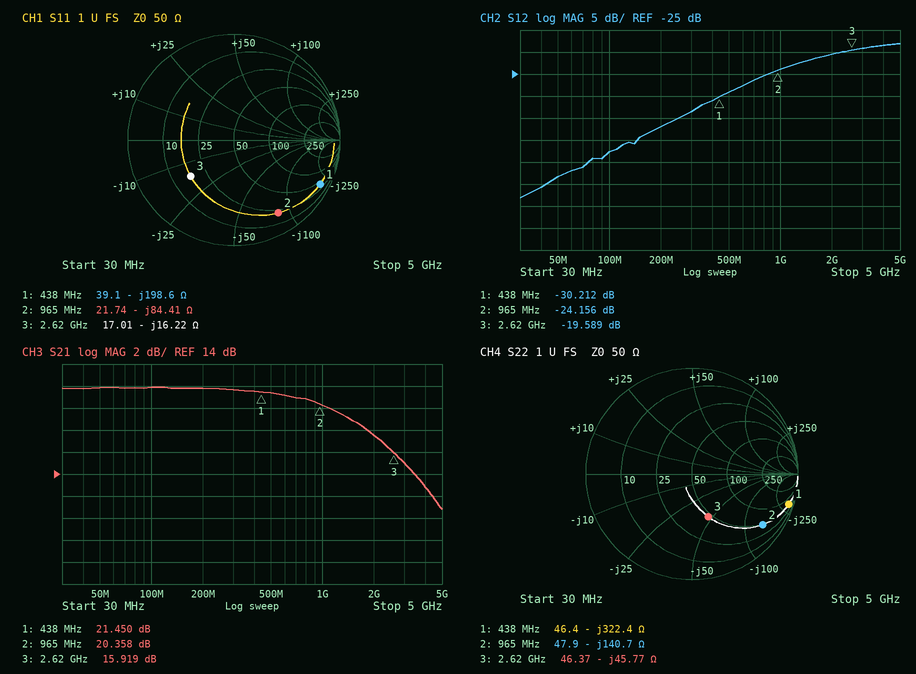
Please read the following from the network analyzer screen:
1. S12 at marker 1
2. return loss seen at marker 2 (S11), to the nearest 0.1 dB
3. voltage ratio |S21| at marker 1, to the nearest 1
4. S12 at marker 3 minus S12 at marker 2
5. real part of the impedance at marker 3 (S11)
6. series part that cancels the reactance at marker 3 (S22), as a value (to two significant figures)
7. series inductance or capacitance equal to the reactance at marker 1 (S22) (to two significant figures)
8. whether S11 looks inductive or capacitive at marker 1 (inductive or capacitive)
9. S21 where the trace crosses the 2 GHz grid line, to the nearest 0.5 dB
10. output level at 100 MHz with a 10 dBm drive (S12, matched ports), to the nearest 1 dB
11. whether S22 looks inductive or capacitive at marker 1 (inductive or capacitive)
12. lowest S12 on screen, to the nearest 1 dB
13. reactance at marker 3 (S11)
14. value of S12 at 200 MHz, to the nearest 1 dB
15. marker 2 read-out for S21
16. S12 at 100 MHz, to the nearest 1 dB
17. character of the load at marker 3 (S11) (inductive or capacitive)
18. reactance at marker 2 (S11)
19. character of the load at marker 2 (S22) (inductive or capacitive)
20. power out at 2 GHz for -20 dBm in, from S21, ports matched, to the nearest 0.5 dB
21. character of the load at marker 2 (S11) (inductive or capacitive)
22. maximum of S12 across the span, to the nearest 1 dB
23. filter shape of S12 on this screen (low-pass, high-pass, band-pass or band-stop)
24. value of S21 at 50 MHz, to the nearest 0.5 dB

-30.212 dB
1.9 dB
12
4.567 dB
17.01 Ω
2.8 nH
1.1 pF
capacitive
17.5 dB
-33 dBm
capacitive
-53 dB
-16.22 Ω
-37 dB
20.358 dB
-43 dB
capacitive
-84.41 Ω
capacitive
-2.5 dBm
capacitive
-18 dB
high-pass
22.0 dB
